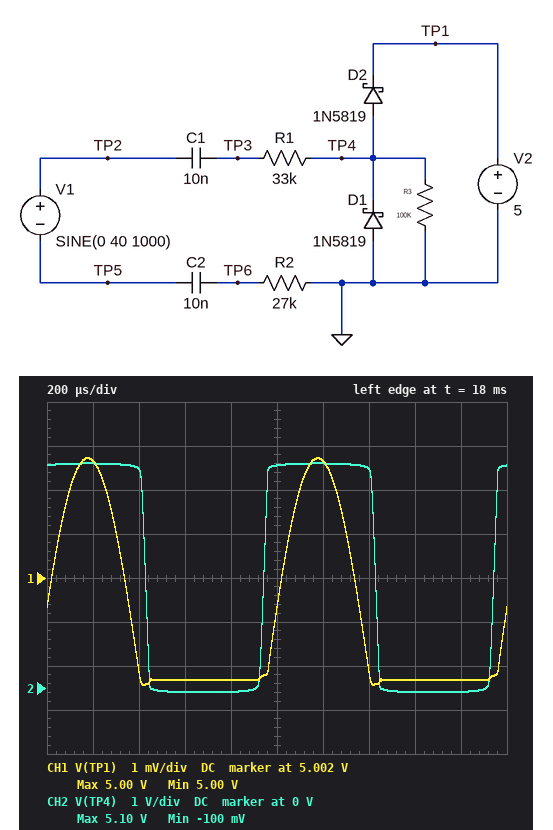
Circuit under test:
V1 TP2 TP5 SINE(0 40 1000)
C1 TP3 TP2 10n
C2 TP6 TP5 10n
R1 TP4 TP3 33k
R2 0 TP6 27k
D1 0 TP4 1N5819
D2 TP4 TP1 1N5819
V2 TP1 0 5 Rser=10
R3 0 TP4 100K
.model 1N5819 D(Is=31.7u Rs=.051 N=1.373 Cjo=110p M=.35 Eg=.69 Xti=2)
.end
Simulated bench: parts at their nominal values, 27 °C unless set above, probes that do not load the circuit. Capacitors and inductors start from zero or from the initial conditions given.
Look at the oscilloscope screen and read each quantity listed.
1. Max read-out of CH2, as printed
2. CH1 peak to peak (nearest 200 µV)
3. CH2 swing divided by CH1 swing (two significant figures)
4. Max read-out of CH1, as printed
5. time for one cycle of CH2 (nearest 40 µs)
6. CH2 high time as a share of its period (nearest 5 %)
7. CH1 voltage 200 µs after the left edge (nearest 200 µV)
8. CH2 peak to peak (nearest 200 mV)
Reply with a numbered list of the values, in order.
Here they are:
1. 5.10 V
2. 5.2 mV
3. 1000
4. 5.00 V
5. 1.00 ms
6. 50 %
7. 5.0046 V
8. 5.2 V
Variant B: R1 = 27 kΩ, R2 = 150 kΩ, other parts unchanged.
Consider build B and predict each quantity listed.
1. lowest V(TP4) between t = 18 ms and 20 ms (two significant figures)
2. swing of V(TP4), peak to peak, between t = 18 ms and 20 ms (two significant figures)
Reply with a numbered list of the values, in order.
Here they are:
1. -67 mV
2. 5.1 V
